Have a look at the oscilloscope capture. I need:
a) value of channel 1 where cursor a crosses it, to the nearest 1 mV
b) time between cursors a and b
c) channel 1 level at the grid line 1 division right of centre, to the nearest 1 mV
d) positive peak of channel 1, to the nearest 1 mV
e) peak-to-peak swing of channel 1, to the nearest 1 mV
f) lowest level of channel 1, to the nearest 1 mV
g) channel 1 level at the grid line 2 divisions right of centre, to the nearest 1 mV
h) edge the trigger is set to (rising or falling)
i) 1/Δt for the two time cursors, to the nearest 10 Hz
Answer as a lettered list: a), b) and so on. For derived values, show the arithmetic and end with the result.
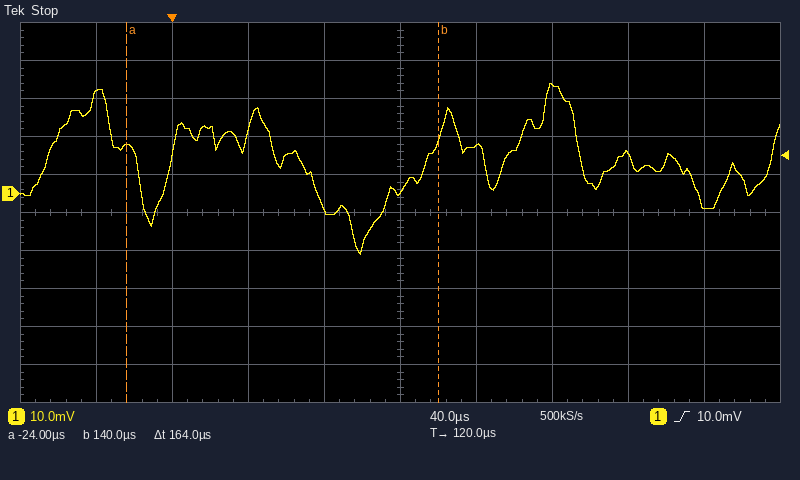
a) 13 mV
b) 164 µs
c) 13 mV
d) 29 mV
e) 29 mV − (-16 mV) = 45 mV
f) -16 mV
g) 28 mV
h) rising
i) 1 / 164 µs ≈ 6.10 kHz
